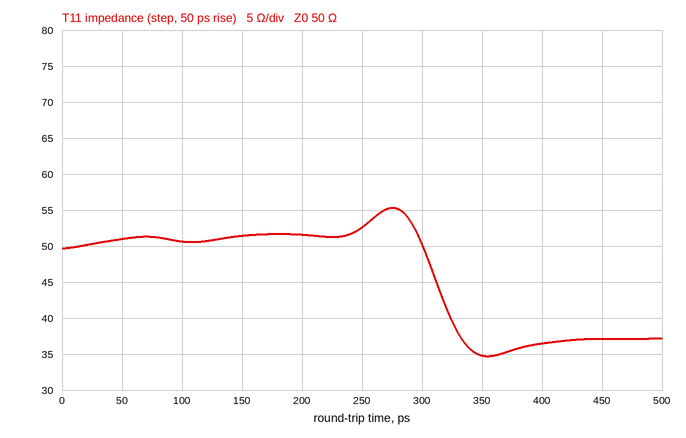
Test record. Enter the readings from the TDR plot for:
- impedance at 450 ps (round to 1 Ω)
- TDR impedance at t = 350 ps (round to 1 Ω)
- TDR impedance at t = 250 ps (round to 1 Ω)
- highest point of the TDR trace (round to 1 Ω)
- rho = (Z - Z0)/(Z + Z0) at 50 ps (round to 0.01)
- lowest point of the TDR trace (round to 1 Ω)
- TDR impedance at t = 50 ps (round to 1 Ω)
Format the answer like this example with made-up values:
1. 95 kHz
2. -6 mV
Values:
1. 37 Ω
2. 35 Ω
3. 53 Ω
4. 55 Ω
5. +0.01
6. 35 Ω
7. 51 Ω
